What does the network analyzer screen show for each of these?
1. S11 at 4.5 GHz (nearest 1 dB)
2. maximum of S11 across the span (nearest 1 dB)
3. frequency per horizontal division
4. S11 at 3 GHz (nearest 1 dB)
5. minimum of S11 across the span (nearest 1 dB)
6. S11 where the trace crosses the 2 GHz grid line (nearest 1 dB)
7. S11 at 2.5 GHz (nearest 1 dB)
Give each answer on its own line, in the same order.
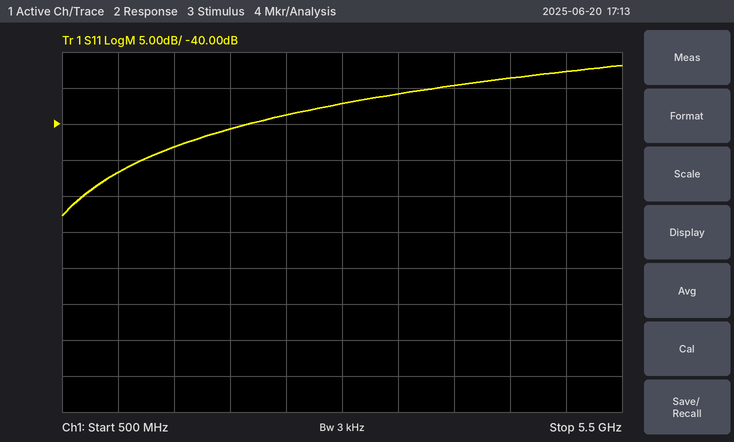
-34 dB
-32 dB
500 MHz
-37 dB
-53 dB
-41 dB
-39 dB
